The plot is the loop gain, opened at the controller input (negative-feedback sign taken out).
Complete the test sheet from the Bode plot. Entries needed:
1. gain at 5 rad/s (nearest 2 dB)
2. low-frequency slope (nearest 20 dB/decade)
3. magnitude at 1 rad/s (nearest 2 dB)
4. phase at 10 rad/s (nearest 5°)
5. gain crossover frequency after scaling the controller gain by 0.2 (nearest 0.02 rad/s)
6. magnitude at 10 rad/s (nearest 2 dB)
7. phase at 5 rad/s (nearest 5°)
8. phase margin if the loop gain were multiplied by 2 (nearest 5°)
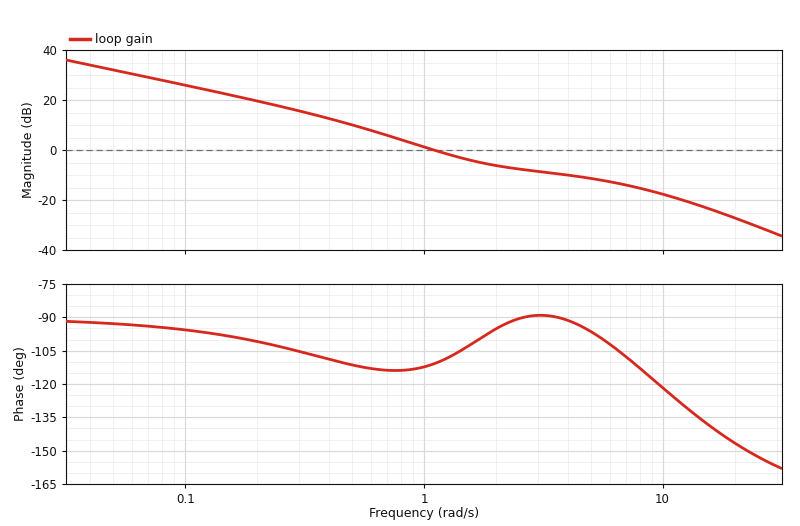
-12 dB
-20 dB/decade
2 dB
-120°
0.36 rad/s
-18 dB
-95°
85°
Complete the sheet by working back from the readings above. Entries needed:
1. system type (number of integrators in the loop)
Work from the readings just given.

1
